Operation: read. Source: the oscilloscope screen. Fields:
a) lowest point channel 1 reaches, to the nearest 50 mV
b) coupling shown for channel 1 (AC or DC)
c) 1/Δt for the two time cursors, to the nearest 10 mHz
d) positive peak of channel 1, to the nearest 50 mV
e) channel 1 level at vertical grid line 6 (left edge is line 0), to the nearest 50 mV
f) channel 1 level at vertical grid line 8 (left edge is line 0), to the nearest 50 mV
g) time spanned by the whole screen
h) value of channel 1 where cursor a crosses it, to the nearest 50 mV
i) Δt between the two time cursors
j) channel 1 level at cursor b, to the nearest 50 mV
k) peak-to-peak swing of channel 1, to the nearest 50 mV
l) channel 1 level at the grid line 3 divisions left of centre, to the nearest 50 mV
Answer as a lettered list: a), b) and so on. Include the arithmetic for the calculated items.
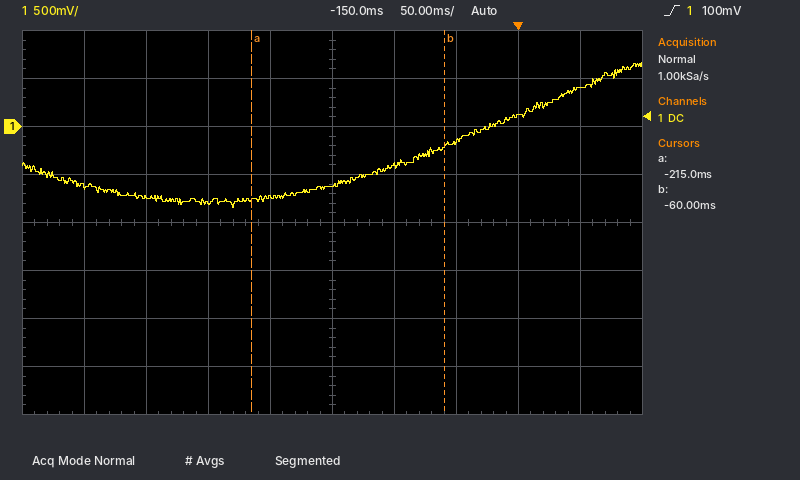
a) -850 mV
b) DC
c) 1 / 155 ms ≈ 6.45 Hz
d) 650 mV
e) -400 mV
f) 100 mV
g) 500 ms
h) -750 mV
i) -60 ms − (-215 ms) = 155 ms
j) -200 mV
k) 650 mV − (-850 mV) = 1.50 V
l) -750 mV
